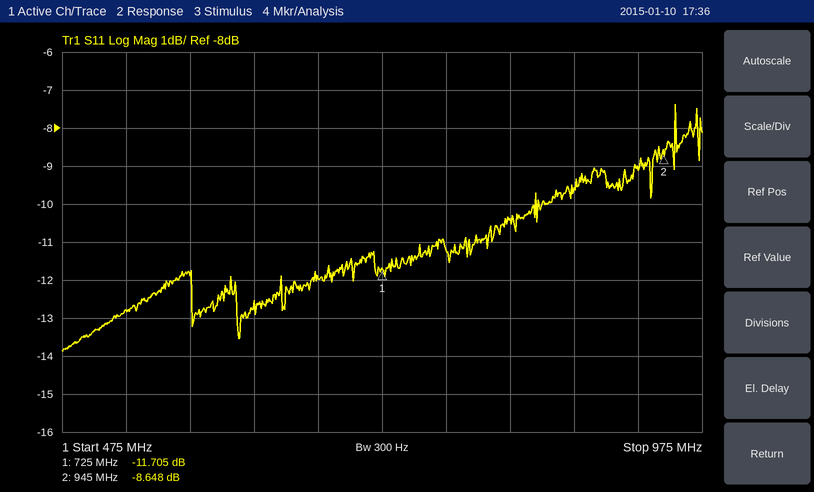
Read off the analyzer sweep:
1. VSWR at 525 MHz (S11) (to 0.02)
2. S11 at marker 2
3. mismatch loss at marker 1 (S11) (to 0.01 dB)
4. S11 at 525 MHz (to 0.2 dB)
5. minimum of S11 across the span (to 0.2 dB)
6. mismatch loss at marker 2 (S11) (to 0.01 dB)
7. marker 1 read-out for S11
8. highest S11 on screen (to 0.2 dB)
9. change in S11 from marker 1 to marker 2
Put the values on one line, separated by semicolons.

1.60; -8.648 dB; 0.30 dB; -12.8 dB; -13.8 dB; 0.64 dB; -11.705 dB; -7.4 dB; 3.057 dB
